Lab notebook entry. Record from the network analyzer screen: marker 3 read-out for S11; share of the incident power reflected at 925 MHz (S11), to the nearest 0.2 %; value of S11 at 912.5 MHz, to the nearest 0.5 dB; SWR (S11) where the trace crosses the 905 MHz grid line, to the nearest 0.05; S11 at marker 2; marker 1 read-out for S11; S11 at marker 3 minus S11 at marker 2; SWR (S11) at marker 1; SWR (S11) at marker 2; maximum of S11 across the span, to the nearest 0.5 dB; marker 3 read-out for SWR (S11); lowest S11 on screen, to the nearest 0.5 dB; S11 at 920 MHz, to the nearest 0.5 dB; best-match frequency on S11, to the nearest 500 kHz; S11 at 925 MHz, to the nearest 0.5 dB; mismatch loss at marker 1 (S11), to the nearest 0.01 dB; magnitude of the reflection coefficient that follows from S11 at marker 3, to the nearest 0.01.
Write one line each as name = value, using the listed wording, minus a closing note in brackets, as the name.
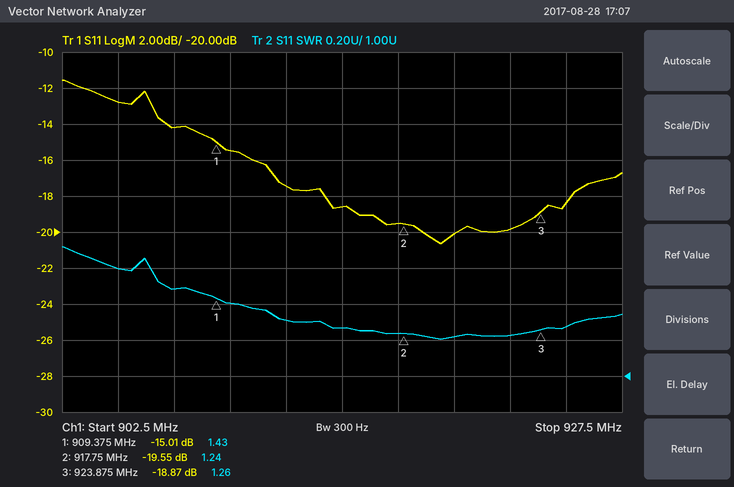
marker 3 read-out for S11 = -18.87 dB
share of the incident power reflected at 925 MHz (S11), to the nearest 0.2 % = 1.4 %
value of S11 at 912.5 MHz, to the nearest 0.5 dB = -17.5 dB
SWR (S11) where the trace crosses the 905 MHz grid line, to the nearest 0.05 = 1.60
S11 at marker 2 = -19.55 dB
marker 1 read-out for S11 = -15.01 dB
S11 at marker 3 minus S11 at marker 2 = 0.68 dB
SWR (S11) at marker 1 = 1.43
SWR (S11) at marker 2 = 1.24
maximum of S11 across the span, to the nearest 0.5 dB = -11.5 dB
marker 3 read-out for SWR = 1.26
lowest S11 on screen, to the nearest 0.5 dB = -20.5 dB
S11 at 920 MHz, to the nearest 0.5 dB = -20.0 dB
best-match frequency on S11, to the nearest 500 kHz = 919.5 MHz
S11 at 925 MHz, to the nearest 0.5 dB = -18.5 dB
mismatch loss at marker 1 (S11), to the nearest 0.01 dB = 0.14 dB
magnitude of the reflection coefficient that follows from S11 at marker 3, to the nearest 0.01 = 0.11
